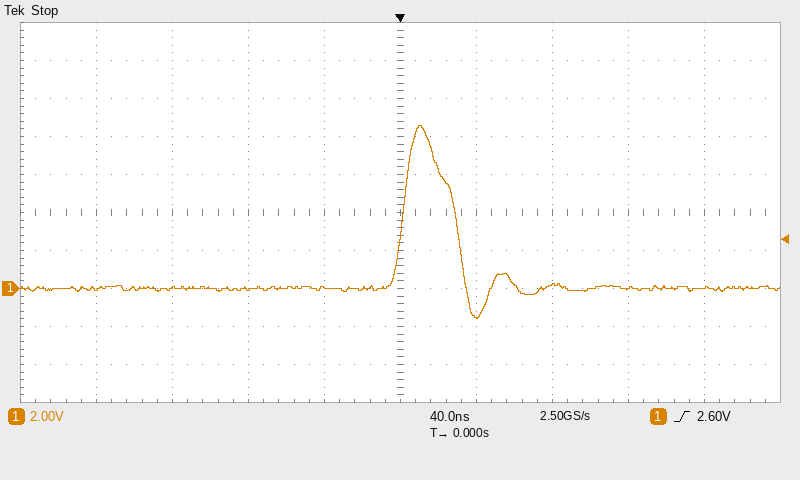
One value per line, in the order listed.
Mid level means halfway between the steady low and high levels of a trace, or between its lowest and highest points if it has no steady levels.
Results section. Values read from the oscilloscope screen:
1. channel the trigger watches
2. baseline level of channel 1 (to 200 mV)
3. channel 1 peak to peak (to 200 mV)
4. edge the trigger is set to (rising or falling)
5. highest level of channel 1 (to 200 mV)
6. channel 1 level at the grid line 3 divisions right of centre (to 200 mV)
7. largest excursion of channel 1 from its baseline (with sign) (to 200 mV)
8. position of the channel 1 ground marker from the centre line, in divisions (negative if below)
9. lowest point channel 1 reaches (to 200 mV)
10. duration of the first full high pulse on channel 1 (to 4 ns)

channel 1
0.0 V
10.2 V
rising
8.6 V
0.0 V
+8.6 V
-2.0 div
-1.6 V
28 ns
